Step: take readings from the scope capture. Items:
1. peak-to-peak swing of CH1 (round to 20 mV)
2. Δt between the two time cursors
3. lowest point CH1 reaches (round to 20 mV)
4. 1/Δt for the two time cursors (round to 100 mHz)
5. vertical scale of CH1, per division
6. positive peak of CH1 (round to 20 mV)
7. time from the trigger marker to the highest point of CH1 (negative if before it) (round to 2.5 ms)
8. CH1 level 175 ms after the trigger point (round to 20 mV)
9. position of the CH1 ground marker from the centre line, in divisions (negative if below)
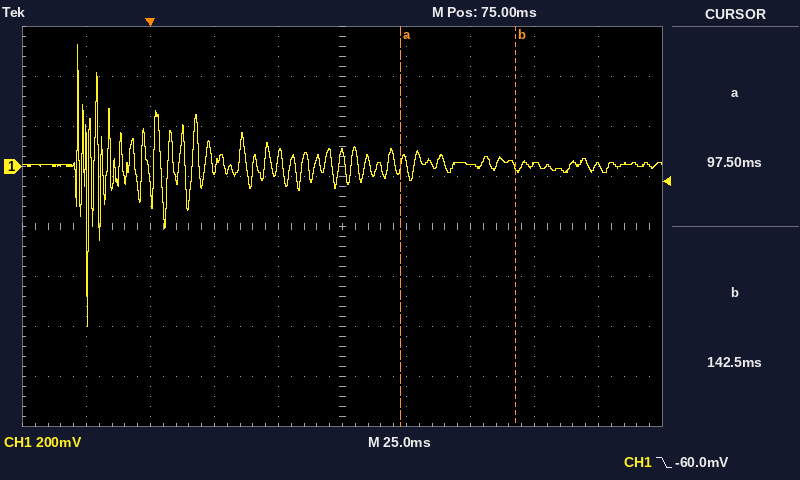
1.12 V
45.0 ms
-640 mV
22.2 Hz
200 mV
480 mV
-27.5 ms
0 mV
+1.2 div
